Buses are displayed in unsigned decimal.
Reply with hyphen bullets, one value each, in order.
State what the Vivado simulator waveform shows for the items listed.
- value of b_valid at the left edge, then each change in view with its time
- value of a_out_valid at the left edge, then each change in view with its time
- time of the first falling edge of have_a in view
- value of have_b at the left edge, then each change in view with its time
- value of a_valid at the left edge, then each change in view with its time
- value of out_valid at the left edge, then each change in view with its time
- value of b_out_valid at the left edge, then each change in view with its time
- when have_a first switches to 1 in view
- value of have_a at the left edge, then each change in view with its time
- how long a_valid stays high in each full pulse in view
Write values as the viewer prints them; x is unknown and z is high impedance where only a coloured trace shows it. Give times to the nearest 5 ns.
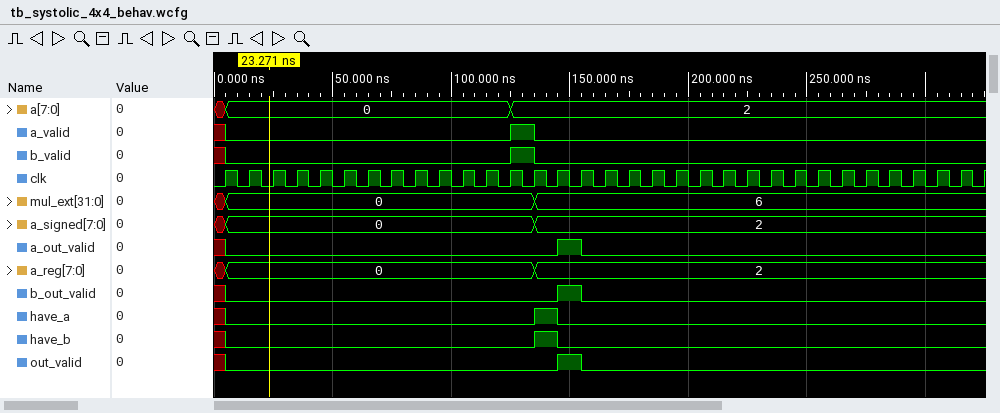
- x, 0 at 5 ns, 1 at 125 ns, 0 at 135 ns
- x, 0 at 5 ns, 1 at 145 ns, 0 at 155 ns
- 145 ns
- x, 0 at 5 ns, 1 at 135 ns, 0 at 145 ns
- x, 0 at 5 ns, 1 at 125 ns, 0 at 135 ns
- x, 0 at 5 ns, 1 at 145 ns, 0 at 155 ns
- x, 0 at 5 ns, 1 at 145 ns, 0 at 155 ns
- 135 ns
- x, 0 at 5 ns, 1 at 135 ns, 0 at 145 ns
- 10 ns
